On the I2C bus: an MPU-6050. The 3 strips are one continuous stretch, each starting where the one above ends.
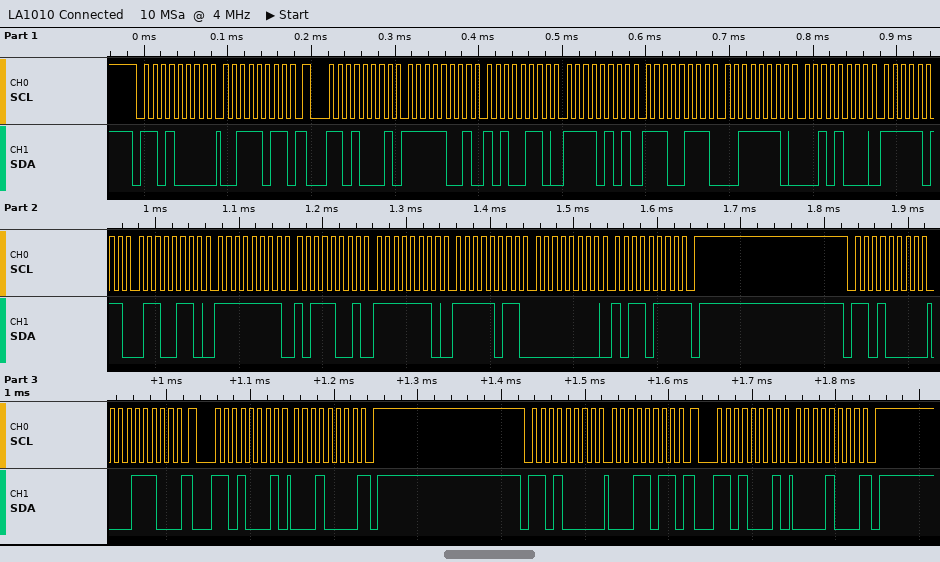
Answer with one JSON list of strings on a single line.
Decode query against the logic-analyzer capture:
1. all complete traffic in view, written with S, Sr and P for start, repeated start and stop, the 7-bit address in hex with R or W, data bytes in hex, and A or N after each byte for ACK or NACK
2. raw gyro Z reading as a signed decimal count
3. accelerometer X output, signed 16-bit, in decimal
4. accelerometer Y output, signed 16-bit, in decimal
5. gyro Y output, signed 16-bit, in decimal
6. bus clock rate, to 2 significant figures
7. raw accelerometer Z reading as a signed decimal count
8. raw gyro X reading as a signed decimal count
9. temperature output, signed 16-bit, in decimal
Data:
["S 68W A 3B A Sr 68R A F9 A A6 A F5 A E7 A 3E A 28 A FB A 66 A FF A B9 A FE A FB A 00 A B7 N P S 68W A 1C A Sr 68R A 10 N P S 68W A 1B A Sr 68R A 08 N P", "183", "-1626", "-2585", "-261", "100 kHz", "15912", "-71", "-1178"]
